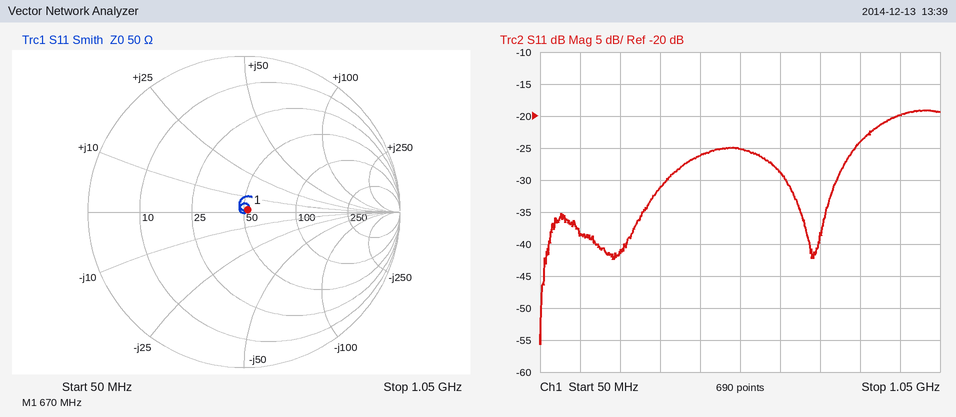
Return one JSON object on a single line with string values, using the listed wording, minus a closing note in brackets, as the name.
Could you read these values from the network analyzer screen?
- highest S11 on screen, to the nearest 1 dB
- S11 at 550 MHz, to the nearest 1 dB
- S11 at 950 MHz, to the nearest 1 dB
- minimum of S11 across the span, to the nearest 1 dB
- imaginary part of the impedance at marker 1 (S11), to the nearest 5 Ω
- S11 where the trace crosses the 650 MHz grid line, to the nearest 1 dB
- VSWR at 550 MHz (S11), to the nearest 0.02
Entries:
{"highest S11 on screen, to the nearest 1 dB": "-19 dB", "S11 at 550 MHz, to the nearest 1 dB": "-25 dB", "S11 at 950 MHz, to the nearest 1 dB": "-20 dB", "minimum of S11 across the span, to the nearest 1 dB": "-56 dB", "imaginary part of the impedance at marker 1 (S11), to the nearest 5 Ω": "0 Ω", "S11 where the trace crosses the 650 MHz grid line, to the nearest 1 dB": "-29 dB", "VSWR at 550 MHz (S11), to the nearest 0.02": "1.12"}
